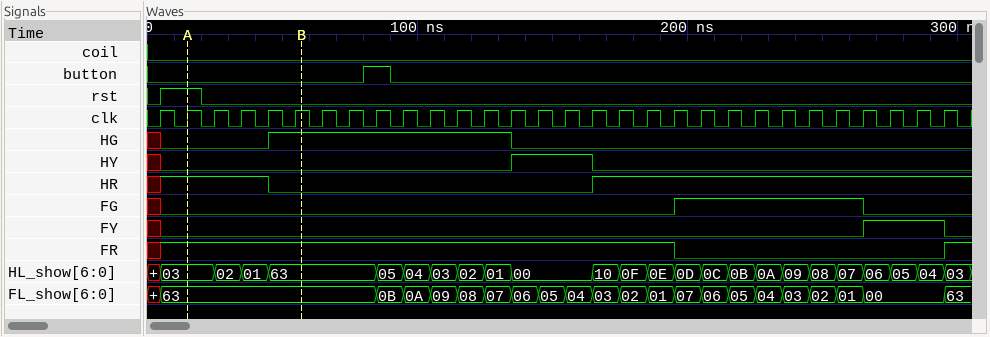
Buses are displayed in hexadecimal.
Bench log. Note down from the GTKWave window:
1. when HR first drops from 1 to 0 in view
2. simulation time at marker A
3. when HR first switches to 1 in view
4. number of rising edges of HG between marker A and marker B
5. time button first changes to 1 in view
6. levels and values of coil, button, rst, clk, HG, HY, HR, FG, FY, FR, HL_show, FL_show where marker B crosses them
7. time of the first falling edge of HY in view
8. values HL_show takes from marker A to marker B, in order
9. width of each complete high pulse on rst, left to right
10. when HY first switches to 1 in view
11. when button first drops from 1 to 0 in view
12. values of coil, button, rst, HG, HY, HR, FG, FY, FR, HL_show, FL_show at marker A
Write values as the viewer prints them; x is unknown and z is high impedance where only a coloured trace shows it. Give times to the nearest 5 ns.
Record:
45 ns
15 ns
5 ns
1
80 ns
coil=0, button=0, rst=0, clk=1, HG=1, HY=0, HR=0, FG=0, FY=0, FR=1, HL_show=63, FL_show=63
165 ns
03, 02, 01, 63
15 ns
135 ns
90 ns
coil=0, button=0, rst=1, HG=0, HY=0, HR=1, FG=0, FY=0, FR=1, HL_show=03, FL_show=63
